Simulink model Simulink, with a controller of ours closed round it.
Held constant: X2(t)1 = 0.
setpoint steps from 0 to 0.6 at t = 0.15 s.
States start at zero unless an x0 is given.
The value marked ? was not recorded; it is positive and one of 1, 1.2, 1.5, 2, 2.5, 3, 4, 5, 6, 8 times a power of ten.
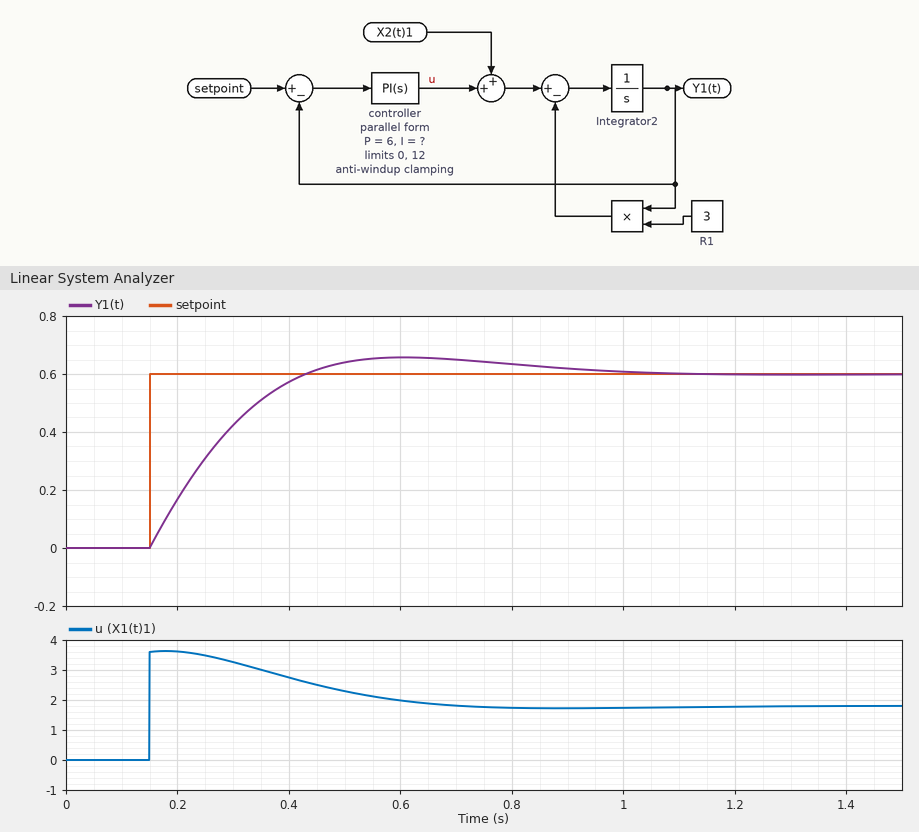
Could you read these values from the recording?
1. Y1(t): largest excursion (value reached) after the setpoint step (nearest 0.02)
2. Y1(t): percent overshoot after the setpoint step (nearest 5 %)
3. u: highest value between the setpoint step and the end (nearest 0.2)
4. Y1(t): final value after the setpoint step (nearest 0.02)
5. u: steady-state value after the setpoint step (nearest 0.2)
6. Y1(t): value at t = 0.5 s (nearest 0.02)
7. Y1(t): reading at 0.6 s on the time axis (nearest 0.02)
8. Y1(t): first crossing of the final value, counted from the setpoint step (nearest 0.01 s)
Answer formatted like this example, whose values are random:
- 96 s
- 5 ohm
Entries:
- 0.66
- 10 %
- 3.6
- 0.60
- 1.8
- 0.64
- 0.66
- 0.28 s
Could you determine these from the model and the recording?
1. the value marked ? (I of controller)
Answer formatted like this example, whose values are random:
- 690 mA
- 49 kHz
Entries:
- 40
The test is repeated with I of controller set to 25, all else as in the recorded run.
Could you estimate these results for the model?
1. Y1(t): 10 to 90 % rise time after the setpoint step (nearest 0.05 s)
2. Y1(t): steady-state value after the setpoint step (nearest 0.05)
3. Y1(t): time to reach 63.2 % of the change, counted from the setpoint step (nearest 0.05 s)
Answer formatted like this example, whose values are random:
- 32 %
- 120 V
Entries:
- 0.30 s
- 0.60
- 0.15 s
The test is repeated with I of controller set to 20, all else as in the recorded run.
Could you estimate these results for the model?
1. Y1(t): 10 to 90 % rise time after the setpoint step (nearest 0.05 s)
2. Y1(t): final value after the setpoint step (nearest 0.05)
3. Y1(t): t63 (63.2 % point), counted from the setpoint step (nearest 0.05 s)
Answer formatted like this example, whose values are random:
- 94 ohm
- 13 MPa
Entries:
- 0.35 s
- 0.60
- 0.15 s
